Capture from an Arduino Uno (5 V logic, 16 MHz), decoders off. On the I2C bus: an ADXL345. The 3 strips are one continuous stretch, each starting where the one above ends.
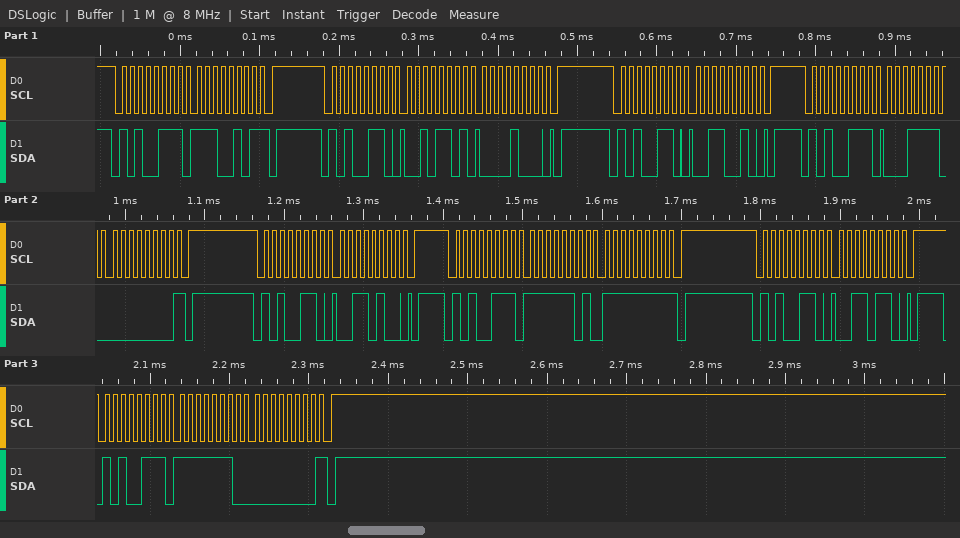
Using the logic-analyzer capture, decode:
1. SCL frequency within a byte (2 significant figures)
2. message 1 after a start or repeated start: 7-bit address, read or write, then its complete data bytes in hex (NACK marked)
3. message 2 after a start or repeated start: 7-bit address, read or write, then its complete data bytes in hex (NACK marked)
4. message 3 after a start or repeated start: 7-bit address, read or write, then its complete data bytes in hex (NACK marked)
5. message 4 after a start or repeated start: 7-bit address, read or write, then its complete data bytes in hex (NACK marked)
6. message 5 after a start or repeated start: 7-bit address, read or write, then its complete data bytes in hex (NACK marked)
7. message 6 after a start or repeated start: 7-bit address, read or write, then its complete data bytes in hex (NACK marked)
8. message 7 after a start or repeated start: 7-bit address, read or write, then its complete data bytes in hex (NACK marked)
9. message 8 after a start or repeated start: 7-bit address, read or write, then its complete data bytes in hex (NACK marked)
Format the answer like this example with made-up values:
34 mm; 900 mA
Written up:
100 kHz; 0x53 read: E5 NACK; 0x53 write: 2D 08; 0x53 write: 32; 0x53 read: 1E 00 NACK; 0x53 write: 34; 0x53 read: FD FF NACK; 0x53 write: 36; 0x53 read: FE 00 NACK
